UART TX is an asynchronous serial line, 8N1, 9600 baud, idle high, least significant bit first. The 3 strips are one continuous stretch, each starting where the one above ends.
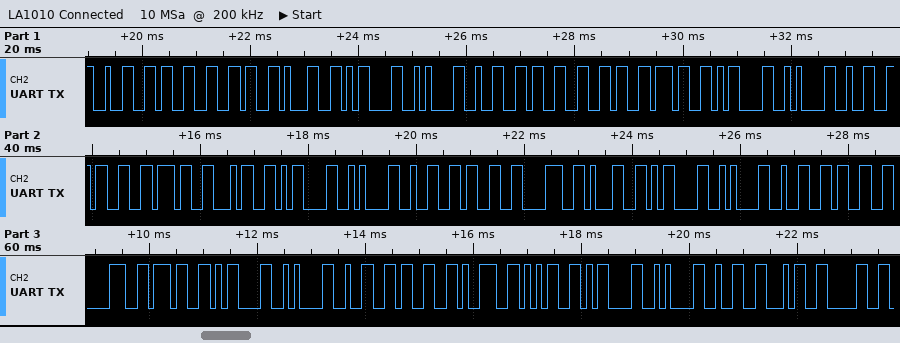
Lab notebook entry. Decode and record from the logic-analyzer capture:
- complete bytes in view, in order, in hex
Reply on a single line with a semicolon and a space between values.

0x32 0x33 0x36 0x31 0x0D 0x0A 0x32 0x33 0x36 0x37 0x0D 0x0A 0x32 0x33 0x37 0x34 0x0D 0x0A 0x32 0x33 0x38 0x31 0x0D 0x0A 0x32 0x33 0x38 0x37 0x0D 0x0A 0x32 0x33 0x39 0x35 0x0D 0x0A 0x32 0x34 0x30
